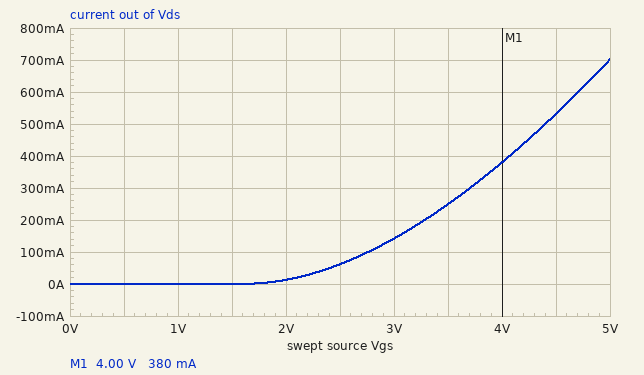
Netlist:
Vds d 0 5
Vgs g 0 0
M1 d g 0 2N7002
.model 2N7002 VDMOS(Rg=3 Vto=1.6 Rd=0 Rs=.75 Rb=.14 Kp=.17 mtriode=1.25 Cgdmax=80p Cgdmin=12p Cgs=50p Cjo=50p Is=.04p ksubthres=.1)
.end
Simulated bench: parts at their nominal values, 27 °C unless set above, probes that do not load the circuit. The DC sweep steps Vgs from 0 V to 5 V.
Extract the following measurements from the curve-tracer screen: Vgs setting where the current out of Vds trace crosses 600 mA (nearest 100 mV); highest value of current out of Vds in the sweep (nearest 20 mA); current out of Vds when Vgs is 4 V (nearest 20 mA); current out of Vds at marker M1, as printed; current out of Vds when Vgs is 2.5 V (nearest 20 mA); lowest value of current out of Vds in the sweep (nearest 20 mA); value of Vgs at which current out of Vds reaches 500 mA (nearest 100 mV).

4.7 V
700 mA
380 mA
380 mA
60 mA
0 A
4.4 V
